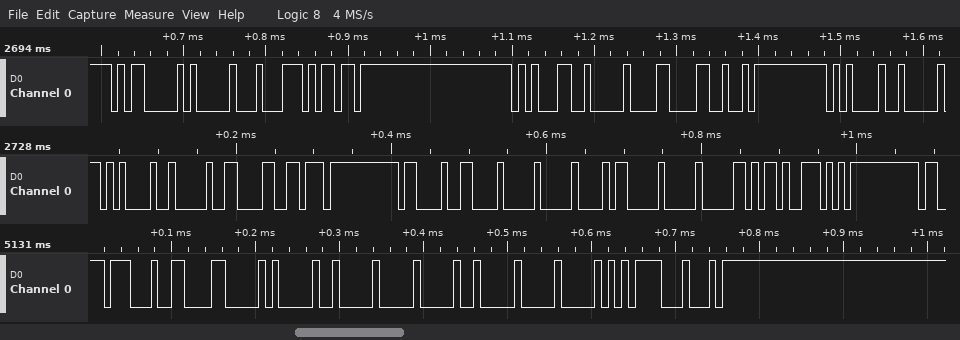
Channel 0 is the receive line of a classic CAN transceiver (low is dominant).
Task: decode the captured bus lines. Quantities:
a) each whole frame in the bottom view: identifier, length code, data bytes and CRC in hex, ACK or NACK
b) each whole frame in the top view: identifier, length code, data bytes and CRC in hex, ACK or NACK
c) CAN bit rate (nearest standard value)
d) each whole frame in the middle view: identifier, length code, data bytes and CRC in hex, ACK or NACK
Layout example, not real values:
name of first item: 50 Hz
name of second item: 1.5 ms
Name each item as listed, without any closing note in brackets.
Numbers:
each whole frame in the bottom view: identifier, length code, data bytes and CRC in hex, ACK or NACK: ID 713, DLC 6, data 04 04 00 01 00 00, CRC 5788, ACK
each whole frame in the top view: identifier, length code, data bytes and CRC in hex, ACK or NACK: ID 581, DLC 0, CRC 23AD, ACK; ID 519, DLC 0, CRC 1864, ACK
CAN bit rate: 125 kbit/s
each whole frame in the middle view: identifier, length code, data bytes and CRC in hex, ACK or NACK: ID 509, DLC 0, CRC 619B, ACK; ID 613, DLC 4, data 00 0B 00 01, CRC 2D3A, ACK
